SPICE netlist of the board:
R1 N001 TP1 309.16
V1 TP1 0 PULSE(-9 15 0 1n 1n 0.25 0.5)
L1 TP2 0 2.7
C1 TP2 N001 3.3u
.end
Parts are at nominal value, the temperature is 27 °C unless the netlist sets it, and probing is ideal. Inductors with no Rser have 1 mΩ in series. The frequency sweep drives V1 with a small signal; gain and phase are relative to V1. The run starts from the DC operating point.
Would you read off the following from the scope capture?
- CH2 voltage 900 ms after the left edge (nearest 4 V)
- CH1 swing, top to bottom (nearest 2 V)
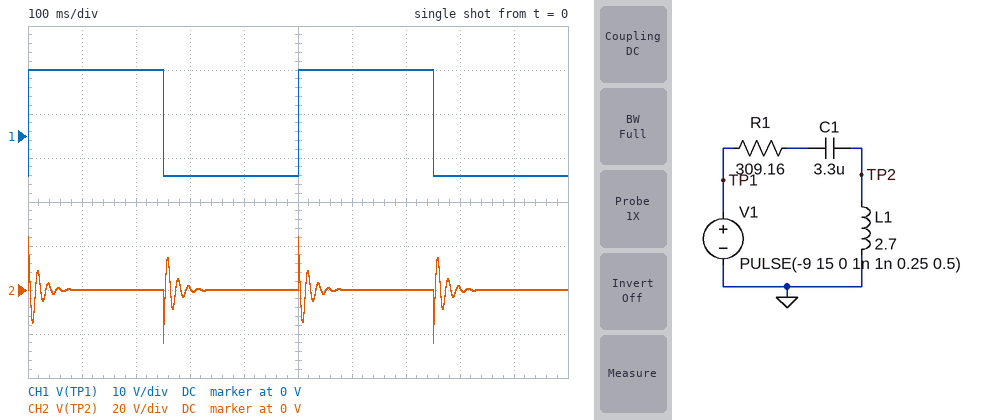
0 V
24 V
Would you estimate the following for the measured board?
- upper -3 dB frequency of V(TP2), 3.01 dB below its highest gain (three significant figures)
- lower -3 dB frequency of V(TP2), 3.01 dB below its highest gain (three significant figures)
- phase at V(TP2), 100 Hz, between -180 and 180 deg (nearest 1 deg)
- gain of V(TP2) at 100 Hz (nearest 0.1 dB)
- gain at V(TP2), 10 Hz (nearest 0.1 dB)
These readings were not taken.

68.6 Hz
47.2 Hz
14 deg
2.6 dB
-28.8 dB
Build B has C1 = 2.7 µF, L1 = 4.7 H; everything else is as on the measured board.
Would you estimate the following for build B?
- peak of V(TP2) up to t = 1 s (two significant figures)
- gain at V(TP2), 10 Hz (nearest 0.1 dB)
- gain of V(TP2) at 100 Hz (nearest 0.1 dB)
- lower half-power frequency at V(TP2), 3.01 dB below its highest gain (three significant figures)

24 V
-25.6 dB
1.9 dB
40.7 Hz
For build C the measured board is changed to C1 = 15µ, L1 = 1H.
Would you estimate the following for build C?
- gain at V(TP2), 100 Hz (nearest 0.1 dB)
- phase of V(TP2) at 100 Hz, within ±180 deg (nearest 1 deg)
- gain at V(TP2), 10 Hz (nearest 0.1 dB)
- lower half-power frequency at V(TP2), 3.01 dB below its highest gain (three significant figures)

0.3 dB
31 deg
-24.4 dB
36.9 Hz
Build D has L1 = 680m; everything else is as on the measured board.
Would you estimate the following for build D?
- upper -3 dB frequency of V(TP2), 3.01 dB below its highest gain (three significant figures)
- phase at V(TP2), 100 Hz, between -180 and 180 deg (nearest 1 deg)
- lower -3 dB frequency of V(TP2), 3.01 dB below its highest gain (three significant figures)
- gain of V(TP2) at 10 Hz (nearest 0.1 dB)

297 Hz
100 deg
89.5 Hz
-41.0 dB
